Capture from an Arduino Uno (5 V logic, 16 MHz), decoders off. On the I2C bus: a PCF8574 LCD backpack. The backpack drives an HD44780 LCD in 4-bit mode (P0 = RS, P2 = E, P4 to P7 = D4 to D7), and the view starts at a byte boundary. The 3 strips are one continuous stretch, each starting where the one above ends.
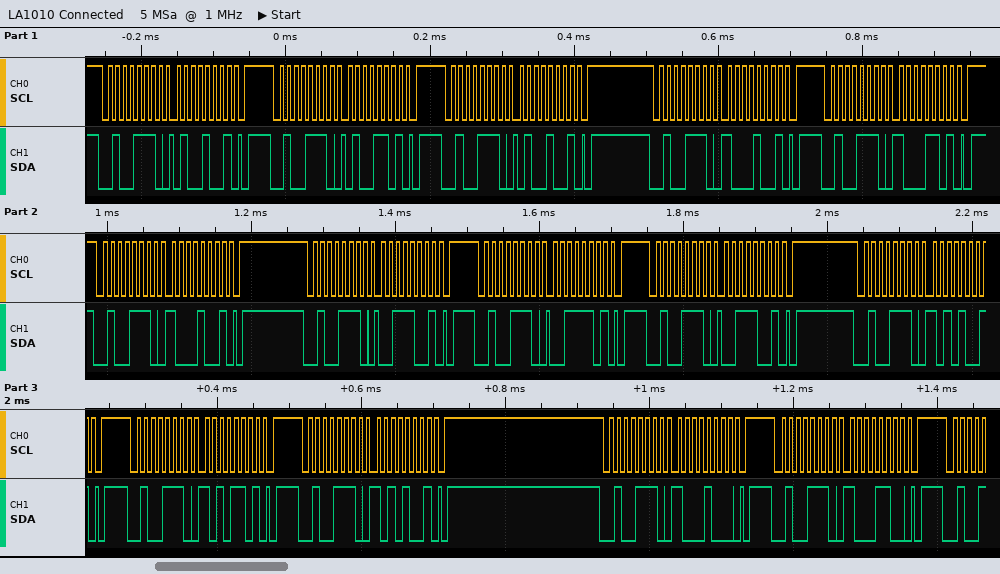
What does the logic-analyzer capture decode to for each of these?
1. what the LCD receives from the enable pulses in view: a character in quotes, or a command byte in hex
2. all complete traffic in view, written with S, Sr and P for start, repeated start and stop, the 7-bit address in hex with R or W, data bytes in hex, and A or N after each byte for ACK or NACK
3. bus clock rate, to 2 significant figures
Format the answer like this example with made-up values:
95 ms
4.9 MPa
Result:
'H' ':'
S 27W A 49 A P S 27W A 4D A P S 27W A 49 A P S 27W A 89 A P S 27W A 8D A P S 27W A 89 A P S 27W A 39 A P S 27W A 3D A P S 27W A 39 A P S 27W A A9 A P S 27W A AD A P S 27W A A9 A P S 27W A 88 A P S 27W A 8C A P
100 kHz
